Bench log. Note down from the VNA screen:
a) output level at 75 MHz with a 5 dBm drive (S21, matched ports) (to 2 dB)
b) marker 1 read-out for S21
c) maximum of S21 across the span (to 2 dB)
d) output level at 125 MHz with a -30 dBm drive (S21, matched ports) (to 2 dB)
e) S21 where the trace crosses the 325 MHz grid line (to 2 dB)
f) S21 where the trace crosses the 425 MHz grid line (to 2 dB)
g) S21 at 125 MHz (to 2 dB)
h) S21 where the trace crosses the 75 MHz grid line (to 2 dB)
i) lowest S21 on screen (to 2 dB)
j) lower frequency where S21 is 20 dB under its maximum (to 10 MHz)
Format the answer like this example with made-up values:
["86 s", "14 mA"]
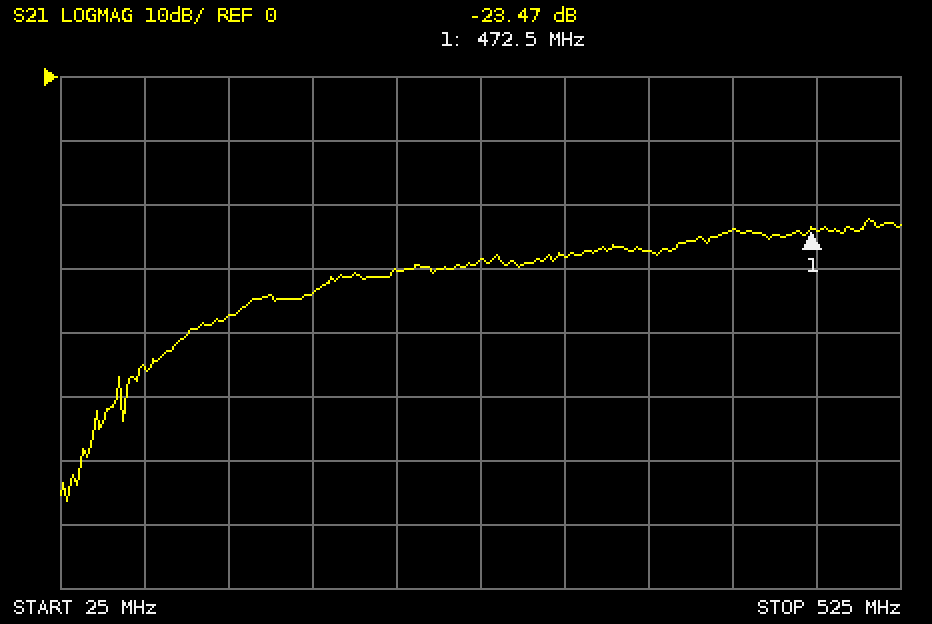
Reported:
["-40 dBm", "-23.47 dB", "-22 dB", "-68 dBm", "-28 dB", "-24 dB", "-38 dB", "-46 dB", "-66 dB", "90 MHz"]
